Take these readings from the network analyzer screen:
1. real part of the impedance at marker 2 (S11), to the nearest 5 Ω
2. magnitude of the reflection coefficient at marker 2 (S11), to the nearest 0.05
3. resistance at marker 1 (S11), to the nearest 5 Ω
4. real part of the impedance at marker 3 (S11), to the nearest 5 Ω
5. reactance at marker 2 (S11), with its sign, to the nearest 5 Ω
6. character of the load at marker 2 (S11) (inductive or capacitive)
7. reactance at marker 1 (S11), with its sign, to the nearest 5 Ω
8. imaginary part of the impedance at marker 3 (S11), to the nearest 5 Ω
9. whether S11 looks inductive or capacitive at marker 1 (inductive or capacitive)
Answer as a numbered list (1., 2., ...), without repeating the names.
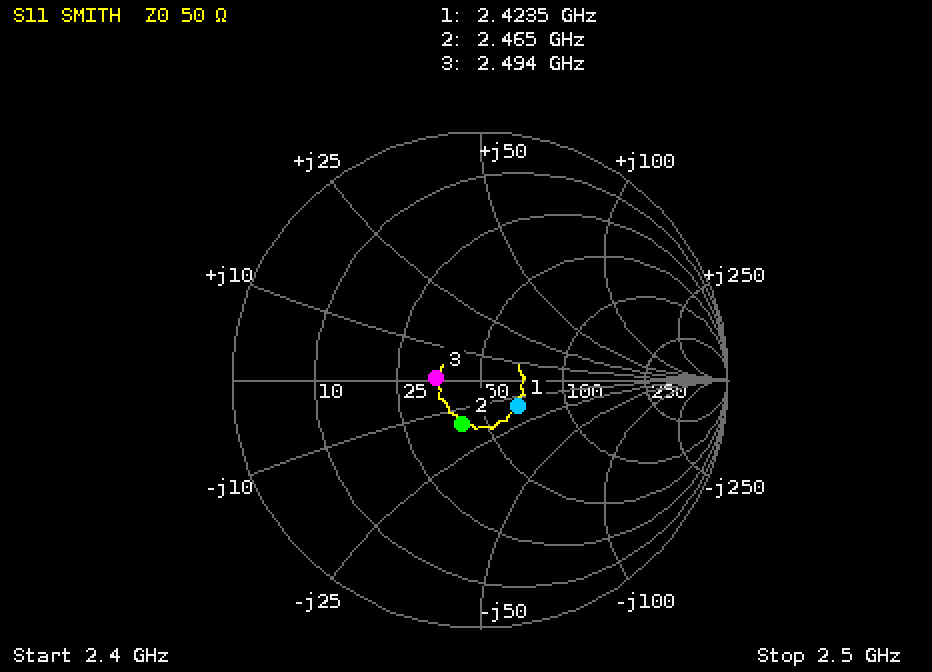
1. 40 Ω
2. 0.20
3. 65 Ω
4. 35 Ω
5. -15 Ω
6. capacitive
7. -15 Ω
8. 0 Ω
9. capacitive
